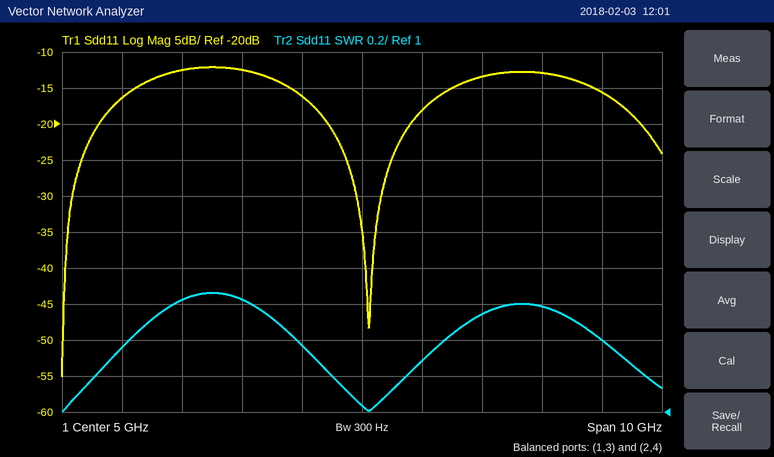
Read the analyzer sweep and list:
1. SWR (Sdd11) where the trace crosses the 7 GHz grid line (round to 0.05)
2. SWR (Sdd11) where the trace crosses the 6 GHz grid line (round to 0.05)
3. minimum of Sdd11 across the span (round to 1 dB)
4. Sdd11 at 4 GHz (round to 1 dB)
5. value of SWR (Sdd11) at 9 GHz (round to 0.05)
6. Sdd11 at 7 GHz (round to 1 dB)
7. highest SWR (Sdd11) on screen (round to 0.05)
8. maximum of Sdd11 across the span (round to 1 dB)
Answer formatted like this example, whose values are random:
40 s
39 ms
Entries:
1.55
1.30
-55 dB
-16 dB
1.40
-13 dB
1.65
-12 dB
